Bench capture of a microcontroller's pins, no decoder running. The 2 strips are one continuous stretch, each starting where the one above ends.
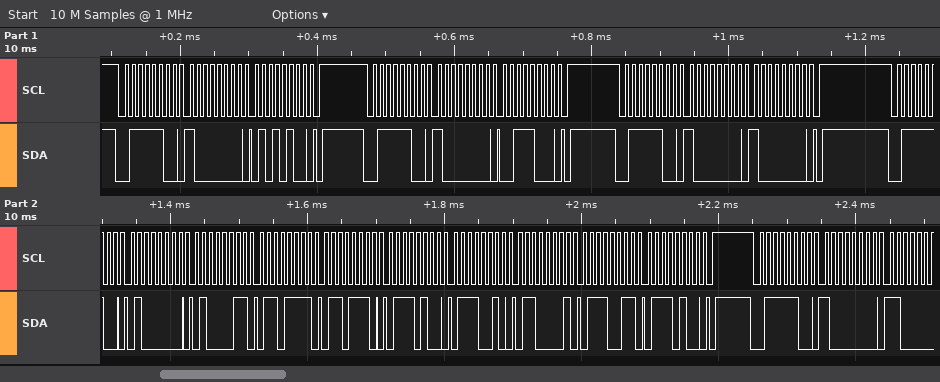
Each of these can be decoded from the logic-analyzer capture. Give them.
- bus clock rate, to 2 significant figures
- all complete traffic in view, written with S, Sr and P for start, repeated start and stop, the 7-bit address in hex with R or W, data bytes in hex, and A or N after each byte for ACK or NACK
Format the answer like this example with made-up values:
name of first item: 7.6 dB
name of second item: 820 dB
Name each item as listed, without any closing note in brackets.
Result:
bus clock rate, to 2 significant figures: 100 kHz
all complete traffic in view, written with S, Sr and P for start, repeated start and stop, the 7-bit address in hex with R or W, data bytes in hex, and A or N after each byte for ACK or NACK: S 3EW A 80 A 54 A P S 3EW A 80 A 38 A P S 3EW A 80 A 80 A P S 3EW A 40 A 43 A 6F A 6E A 74 A 72 A 61 A 73 A 74 A P S 3EW A 80 A
